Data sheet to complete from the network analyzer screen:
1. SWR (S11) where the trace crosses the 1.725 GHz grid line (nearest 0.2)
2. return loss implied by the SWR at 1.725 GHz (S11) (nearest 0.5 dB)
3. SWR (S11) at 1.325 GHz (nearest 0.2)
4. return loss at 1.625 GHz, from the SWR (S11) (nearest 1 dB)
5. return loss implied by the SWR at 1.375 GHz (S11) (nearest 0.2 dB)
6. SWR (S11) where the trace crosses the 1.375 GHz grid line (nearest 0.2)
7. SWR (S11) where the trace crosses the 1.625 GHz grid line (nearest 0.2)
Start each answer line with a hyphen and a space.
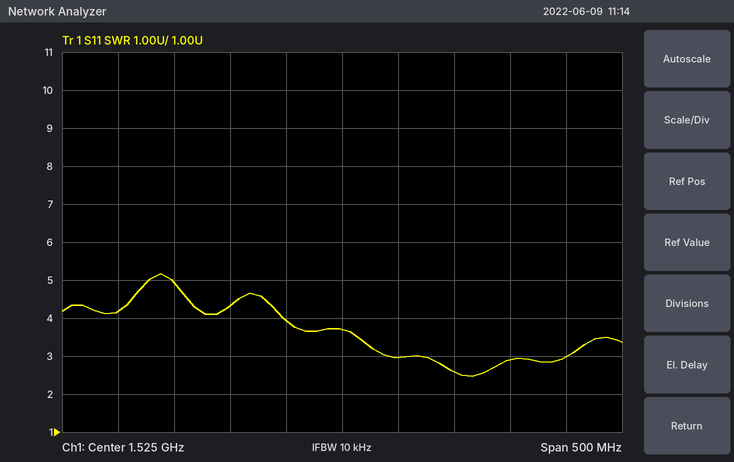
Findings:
- 3.0
- 6.0 dB
- 4.2
- 7 dB
- 3.6 dB
- 5.0
- 2.6
